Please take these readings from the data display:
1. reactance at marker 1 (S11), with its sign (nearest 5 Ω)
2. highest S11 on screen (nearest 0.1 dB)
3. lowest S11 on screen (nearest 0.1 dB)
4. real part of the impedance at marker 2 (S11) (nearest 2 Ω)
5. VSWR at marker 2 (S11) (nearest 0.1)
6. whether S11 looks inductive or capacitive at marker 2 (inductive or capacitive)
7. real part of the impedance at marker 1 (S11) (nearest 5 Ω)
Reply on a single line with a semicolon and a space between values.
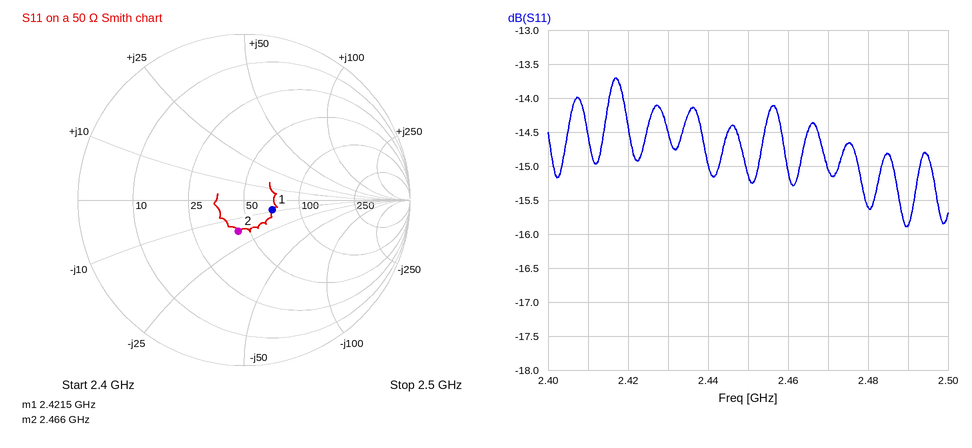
-10 Ω; -13.7 dB; -15.9 dB; 44 Ω; 1.5; capacitive; 70 Ω
